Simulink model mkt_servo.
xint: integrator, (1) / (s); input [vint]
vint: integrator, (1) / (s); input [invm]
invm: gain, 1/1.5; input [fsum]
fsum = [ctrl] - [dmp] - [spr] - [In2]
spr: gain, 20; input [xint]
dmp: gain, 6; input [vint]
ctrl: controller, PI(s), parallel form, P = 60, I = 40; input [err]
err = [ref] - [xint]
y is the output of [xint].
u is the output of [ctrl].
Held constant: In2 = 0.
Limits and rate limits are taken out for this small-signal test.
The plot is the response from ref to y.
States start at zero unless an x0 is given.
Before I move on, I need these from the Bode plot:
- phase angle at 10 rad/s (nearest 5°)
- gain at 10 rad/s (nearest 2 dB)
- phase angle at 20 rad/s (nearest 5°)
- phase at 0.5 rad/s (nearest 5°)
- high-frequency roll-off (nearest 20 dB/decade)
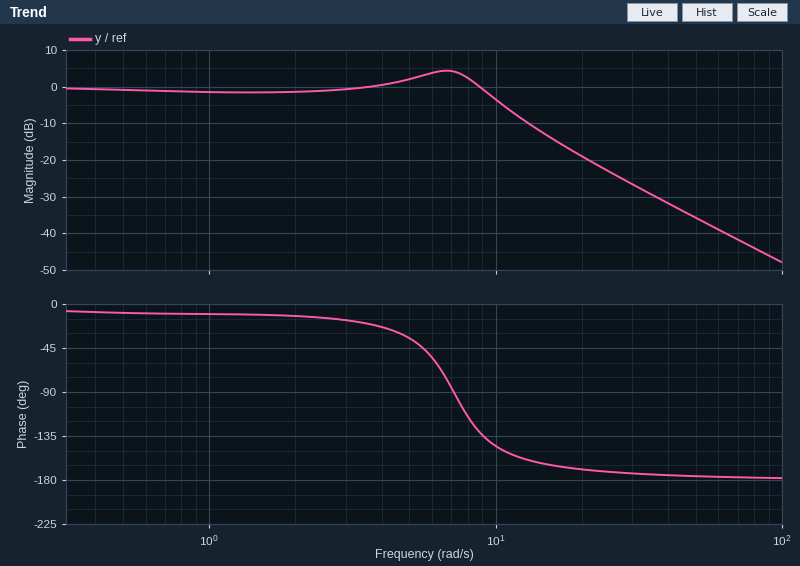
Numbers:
-145°
-4 dB
-170°
-10°
-40 dB/decade
